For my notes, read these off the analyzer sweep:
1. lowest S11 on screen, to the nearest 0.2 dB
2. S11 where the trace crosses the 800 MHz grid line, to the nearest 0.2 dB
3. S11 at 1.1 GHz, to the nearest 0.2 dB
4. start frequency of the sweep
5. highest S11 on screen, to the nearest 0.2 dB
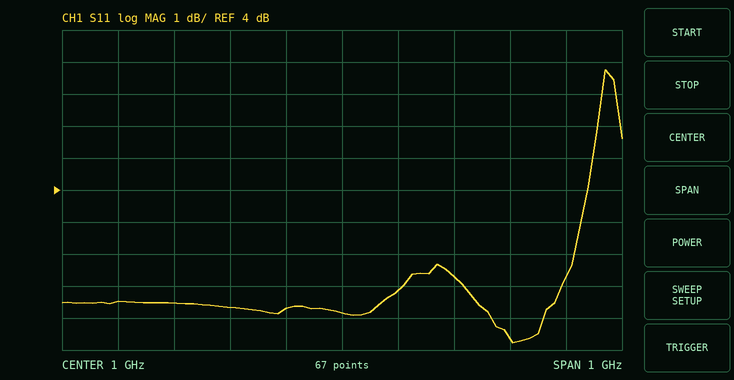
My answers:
-0.8 dB
0.4 dB
0.8 dB
500 MHz
7.8 dB
